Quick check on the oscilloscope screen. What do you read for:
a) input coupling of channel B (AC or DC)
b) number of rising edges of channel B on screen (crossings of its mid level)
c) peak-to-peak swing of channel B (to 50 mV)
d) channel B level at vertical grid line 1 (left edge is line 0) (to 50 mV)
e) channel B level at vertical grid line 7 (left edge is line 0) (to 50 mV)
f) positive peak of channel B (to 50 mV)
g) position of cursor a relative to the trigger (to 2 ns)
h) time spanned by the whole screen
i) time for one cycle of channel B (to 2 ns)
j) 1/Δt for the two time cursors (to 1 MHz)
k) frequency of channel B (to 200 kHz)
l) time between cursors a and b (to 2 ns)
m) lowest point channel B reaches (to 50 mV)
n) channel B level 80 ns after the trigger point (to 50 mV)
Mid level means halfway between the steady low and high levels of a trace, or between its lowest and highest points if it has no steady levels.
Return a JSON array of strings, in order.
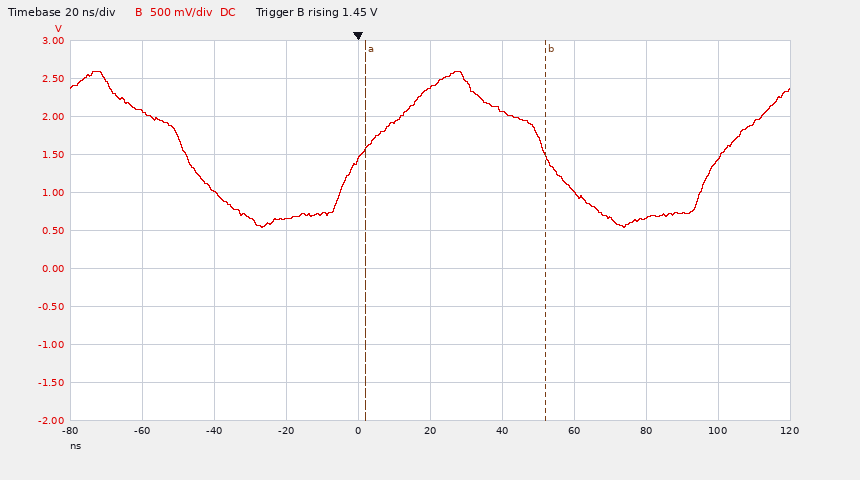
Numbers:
["DC", "2", "2.05 V", "2.05 V", "1.00 V", "2.60 V", "+2 ns", "200 ns", "100 ns", "20 MHz", "10.0 MHz", "50 ns", "550 mV", "650 mV"]
